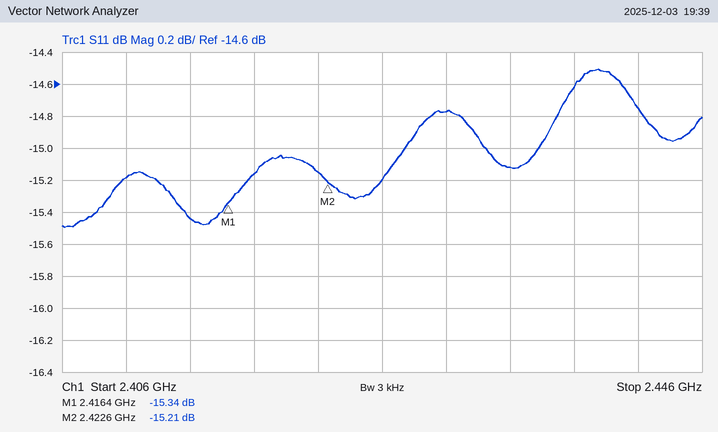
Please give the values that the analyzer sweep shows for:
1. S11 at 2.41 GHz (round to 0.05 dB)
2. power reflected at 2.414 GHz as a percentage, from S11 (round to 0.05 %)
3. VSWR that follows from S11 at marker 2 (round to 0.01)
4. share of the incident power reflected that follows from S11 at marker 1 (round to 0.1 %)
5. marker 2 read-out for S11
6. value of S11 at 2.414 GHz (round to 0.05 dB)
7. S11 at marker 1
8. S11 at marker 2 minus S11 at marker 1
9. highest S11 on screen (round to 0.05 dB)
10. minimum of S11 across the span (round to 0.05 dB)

-15.20 dB
2.85 %
1.42
2.9 %
-15.21 dB
-15.45 dB
-15.34 dB
0.13 dB
-14.50 dB
-15.50 dB
